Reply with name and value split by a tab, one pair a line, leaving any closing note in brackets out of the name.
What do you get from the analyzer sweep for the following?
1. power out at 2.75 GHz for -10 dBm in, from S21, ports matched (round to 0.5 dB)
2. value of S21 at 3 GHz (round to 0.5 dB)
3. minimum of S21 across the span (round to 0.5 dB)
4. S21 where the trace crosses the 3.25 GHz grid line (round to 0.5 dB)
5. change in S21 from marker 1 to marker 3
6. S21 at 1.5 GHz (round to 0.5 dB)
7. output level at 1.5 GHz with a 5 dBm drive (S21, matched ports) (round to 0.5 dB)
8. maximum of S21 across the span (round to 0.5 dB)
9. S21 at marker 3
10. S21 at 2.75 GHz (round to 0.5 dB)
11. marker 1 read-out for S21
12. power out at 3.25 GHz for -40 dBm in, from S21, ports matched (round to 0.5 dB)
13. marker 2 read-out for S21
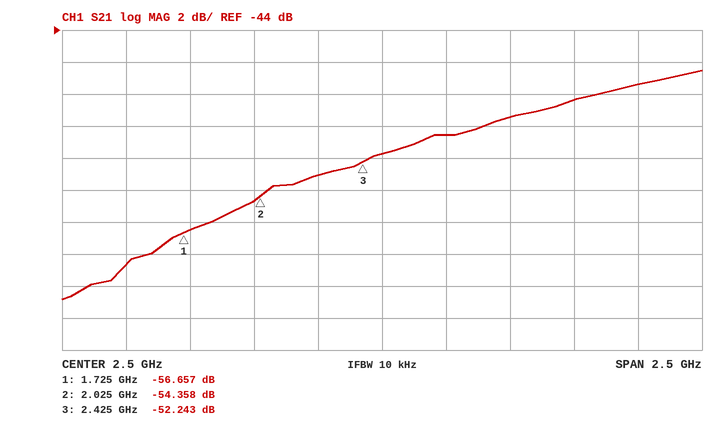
power out at 2.75 GHz for -10 dBm in, from S21, ports matched	-60.5 dBm
value of S21 at 3 GHz	-49.5 dB
minimum of S21 across the span	-61.0 dB
S21 where the trace crosses the 3.25 GHz grid line	-48.5 dB
change in S21 from marker 1 to marker 3	4.414 dB
S21 at 1.5 GHz	-58.5 dB
output level at 1.5 GHz with a 5 dBm drive (S21, matched ports)	-53.5 dBm
maximum of S21 across the span	-46.5 dB
S21 at marker 3	-52.243 dB
S21 at 2.75 GHz	-50.5 dB
marker 1 read-out for S21	-56.657 dB
power out at 3.25 GHz for -40 dBm in, from S21, ports matched	-88.5 dBm
marker 2 read-out for S21	-54.358 dB
